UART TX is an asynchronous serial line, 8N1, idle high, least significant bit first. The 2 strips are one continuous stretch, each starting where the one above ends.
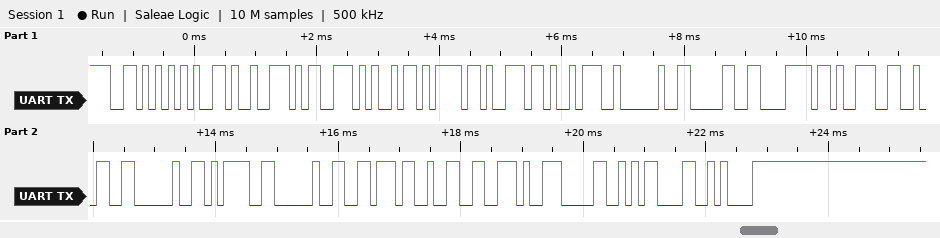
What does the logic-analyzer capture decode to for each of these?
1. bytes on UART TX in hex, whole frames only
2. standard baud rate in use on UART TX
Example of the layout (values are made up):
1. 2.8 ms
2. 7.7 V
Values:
1. 0x56 0x65 0x72 0x73 0x69 0x6F 0x6E 0x3A 0x20 0x30 0x78 0x39 0x32 0x20 0x3D 0x20 0x76 0x32 0x2E 0x30 0x0D 0x0A
2. 9600 baud
